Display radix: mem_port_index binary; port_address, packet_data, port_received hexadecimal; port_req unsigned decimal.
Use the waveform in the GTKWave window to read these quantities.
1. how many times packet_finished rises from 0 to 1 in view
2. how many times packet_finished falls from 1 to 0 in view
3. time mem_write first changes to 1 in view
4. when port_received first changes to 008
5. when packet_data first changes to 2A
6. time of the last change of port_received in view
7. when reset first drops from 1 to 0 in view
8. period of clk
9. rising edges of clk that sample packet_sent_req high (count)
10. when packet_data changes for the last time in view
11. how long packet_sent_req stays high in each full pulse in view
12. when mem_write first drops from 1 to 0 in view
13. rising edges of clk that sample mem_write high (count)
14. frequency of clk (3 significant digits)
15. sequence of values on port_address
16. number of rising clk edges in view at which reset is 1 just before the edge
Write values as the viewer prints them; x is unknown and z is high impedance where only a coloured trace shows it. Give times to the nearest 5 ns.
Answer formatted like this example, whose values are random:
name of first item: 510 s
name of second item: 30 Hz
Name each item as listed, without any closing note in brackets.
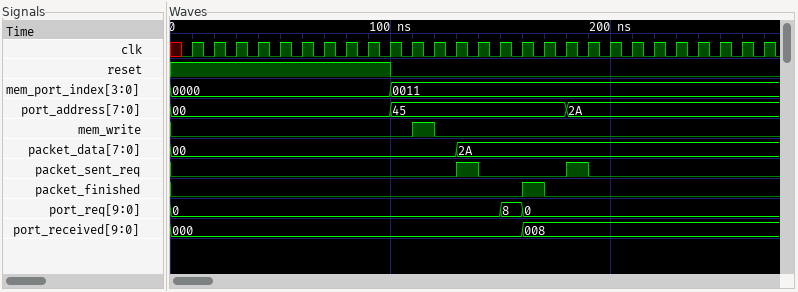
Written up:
how many times packet_finished rises from 0 to 1 in view: 1
how many times packet_finished falls from 1 to 0 in view: 1
time mem_write first changes to 1 in view: 110 ns
when port_received first changes to 008: 160 ns
when packet_data first changes to 2A: 130 ns
time of the last change of port_received in view: 160 ns
when reset first drops from 1 to 0 in view: 100 ns
period of clk: 10 ns
rising edges of clk that sample packet_sent_req high: 2
when packet_data changes for the last time in view: 130 ns
how long packet_sent_req stays high in each full pulse in view: 10 ns, 10 ns
when mem_write first drops from 1 to 0 in view: 120 ns
rising edges of clk that sample mem_write high: 1
frequency of clk: 100 MHz
sequence of values on port_address: 00, 45, 2A
number of rising clk edges in view at which reset is 1 just before the edge: 10
